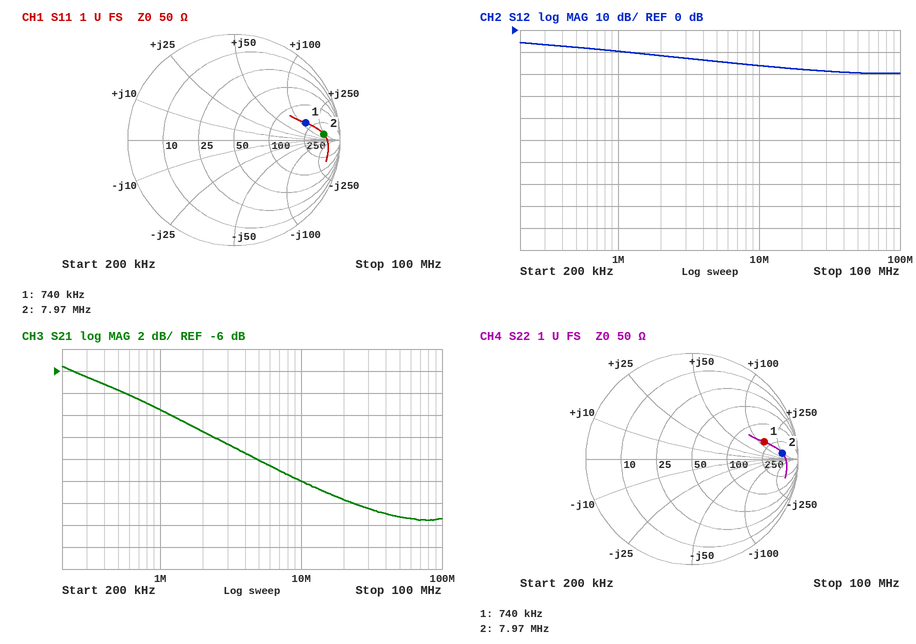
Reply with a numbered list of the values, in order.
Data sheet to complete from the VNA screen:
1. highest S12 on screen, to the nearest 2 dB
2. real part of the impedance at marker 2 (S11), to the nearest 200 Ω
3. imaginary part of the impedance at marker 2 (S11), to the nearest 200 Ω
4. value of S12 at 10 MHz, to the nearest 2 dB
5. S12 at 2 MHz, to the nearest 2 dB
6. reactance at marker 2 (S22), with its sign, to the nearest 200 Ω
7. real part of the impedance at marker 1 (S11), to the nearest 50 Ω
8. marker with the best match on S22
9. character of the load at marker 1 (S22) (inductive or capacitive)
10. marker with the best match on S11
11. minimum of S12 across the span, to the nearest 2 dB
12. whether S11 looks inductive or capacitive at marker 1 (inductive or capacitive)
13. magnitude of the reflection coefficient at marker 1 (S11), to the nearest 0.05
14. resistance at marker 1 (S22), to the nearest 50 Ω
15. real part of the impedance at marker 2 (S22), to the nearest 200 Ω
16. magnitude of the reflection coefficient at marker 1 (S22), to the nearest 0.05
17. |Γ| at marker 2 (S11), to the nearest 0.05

1. -6 dB
2. 600 Ω
3. +200 Ω
4. -16 dB
5. -12 dB
6. +200 Ω
7. 200 Ω
8. marker 1
9. inductive
10. marker 1
11. -20 dB
12. inductive
13. 0.70
14. 200 Ω
15. 600 Ω
16. 0.70
17. 0.85
